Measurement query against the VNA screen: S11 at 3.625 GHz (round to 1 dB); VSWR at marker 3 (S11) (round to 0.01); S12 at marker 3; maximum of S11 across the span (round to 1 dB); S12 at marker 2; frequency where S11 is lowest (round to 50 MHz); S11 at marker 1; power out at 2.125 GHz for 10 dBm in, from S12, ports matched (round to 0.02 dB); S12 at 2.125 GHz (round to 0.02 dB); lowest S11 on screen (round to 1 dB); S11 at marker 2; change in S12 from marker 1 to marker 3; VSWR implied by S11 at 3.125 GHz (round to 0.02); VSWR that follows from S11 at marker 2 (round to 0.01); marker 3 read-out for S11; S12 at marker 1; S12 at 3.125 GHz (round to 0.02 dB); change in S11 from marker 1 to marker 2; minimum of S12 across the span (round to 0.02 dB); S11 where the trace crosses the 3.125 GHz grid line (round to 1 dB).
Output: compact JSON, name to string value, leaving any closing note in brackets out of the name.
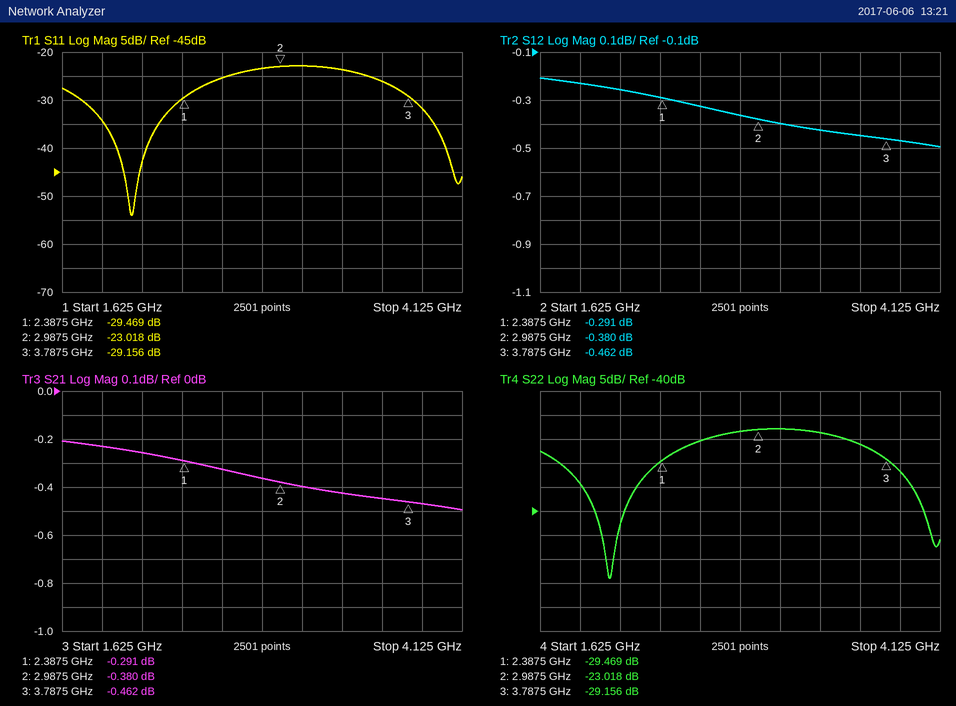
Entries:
{"S11 at 3.625 GHz": "-26 dB", "VSWR at marker 3 (S11)": "1.07", "S12 at marker 3": "-0.462 dB", "maximum of S11 across the span": "-23 dB", "S12 at marker 2": "-0.380 dB", "frequency where S11 is lowest": "2.05 GHz", "S11 at marker 1": "-29.469 dB", "power out at 2.125 GHz for 10 dBm in, from S12, ports matched": "9.74 dBm", "S12 at 2.125 GHz": "-0.26 dB", "lowest S11 on screen": "-54 dB", "S11 at marker 2": "-23.018 dB", "change in S12 from marker 1 to marker 3": "-0.171 dB", "VSWR implied by S11 at 3.125 GHz": "1.16", "VSWR that follows from S11 at marker 2": "1.15", "marker 3 read-out for S11": "-29.156 dB", "S12 at marker 1": "-0.291 dB", "S12 at 3.125 GHz": "-0.40 dB", "change in S11 from marker 1 to marker 2": "6.451 dB", "minimum of S12 across the span": "-0.50 dB", "S11 where the trace crosses the 3.125 GHz grid line": "-23 dB"}
